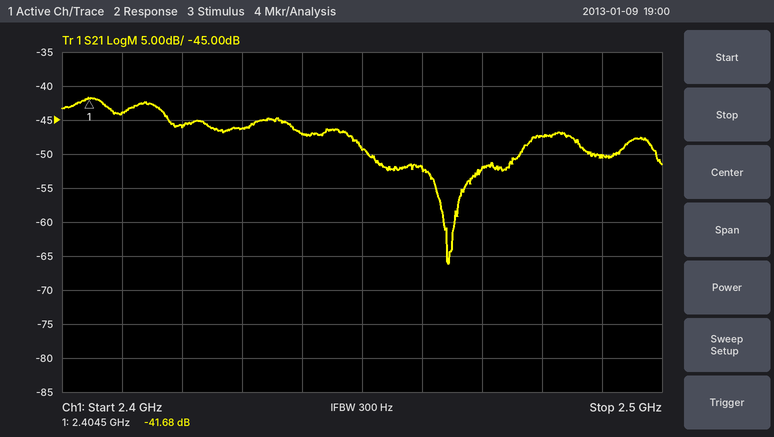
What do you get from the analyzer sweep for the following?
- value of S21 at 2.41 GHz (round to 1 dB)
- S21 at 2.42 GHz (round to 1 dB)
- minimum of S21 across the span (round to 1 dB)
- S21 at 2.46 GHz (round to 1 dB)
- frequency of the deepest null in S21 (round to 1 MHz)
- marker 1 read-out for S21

-44 dB
-46 dB
-66 dB
-52 dB
2.464 GHz
-41.68 dB
